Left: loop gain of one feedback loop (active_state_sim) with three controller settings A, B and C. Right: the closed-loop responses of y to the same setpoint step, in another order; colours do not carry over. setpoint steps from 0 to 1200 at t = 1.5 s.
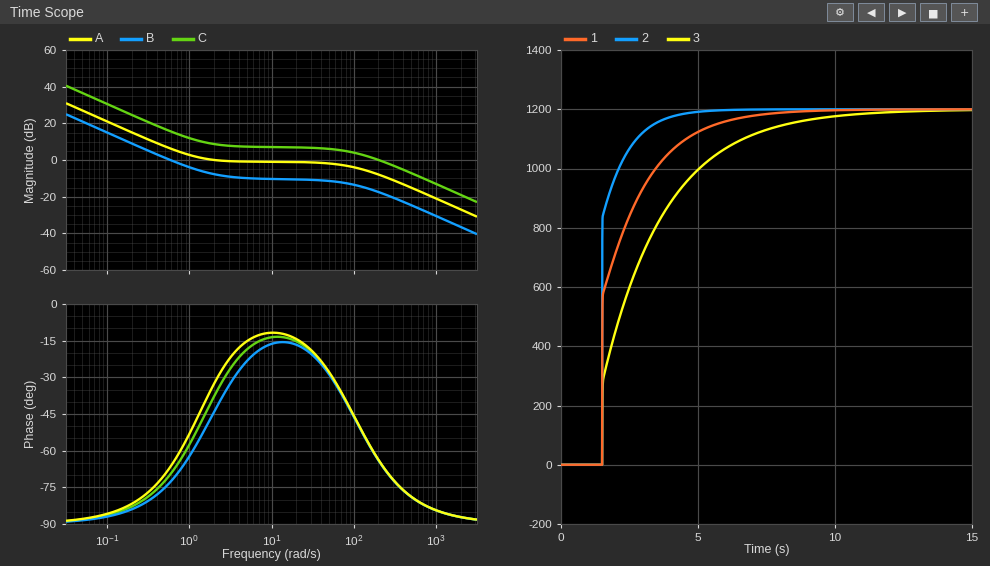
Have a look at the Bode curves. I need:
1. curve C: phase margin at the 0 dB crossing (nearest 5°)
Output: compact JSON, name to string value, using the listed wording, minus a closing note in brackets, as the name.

{"curve C: phase margin at the 0 dB crossing": "115°"}
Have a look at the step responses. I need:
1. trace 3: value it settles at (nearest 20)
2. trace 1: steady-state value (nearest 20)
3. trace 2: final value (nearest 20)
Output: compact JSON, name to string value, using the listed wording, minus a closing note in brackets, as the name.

{"trace 3: value it settles at": "1200", "trace 1: steady-state value": "1200", "trace 2: final value": "1200"}
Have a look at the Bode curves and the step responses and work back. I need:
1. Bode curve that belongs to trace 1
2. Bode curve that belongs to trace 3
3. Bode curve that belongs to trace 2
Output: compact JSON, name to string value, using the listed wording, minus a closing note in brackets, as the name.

{"Bode curve that belongs to trace 1": "A", "Bode curve that belongs to trace 3": "B", "Bode curve that belongs to trace 2": "C"}
